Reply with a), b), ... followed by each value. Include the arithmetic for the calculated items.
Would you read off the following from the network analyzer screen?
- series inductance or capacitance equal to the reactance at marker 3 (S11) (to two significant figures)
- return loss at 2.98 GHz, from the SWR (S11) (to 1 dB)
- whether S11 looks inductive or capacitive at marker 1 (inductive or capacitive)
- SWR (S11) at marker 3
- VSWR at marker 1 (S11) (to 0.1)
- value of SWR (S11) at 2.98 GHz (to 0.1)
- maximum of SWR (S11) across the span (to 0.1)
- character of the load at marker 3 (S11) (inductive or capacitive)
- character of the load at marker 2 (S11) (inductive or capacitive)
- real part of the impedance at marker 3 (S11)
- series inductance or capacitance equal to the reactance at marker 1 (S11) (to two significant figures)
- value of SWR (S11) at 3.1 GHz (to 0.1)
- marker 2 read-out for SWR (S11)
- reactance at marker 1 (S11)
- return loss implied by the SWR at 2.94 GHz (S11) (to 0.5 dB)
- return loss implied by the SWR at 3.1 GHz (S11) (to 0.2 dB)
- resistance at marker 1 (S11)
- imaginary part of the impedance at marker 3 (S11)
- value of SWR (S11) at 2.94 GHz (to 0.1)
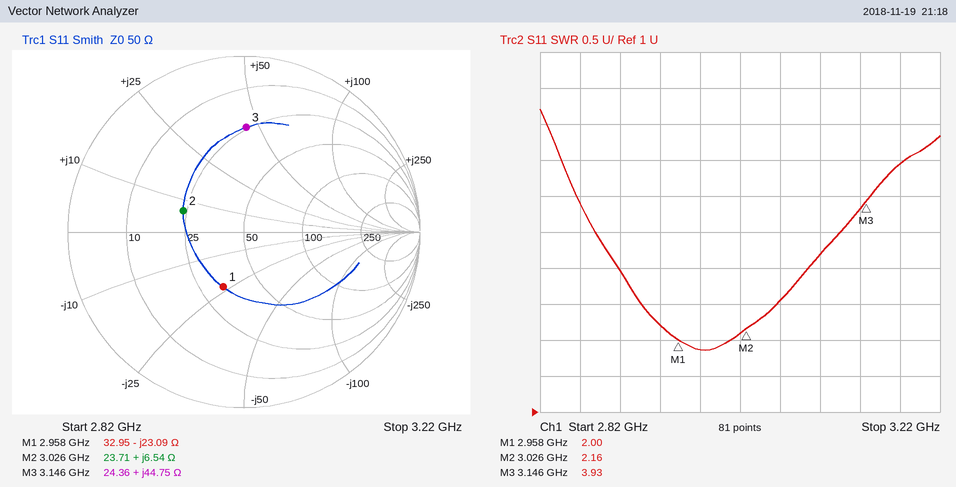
a) L = 44.75 Ω/(2π × 3.146 GHz) ≈ 2.3 nH
b) −20 log10((1.9 − 1)/(1.9 + 1)) ≈ 10 dB
c) capacitive
d) 3.93
e) 2.0
f) 1.9
g) 5.2
h) inductive
i) inductive
j) 24.36 Ω
k) C = 1/(2π × 2.958 GHz × 23.09 Ω) ≈ 2.3 pF
l) 3.2
m) 2.16
n) -23.09 Ω
o) −20 log10((2.2 − 1)/(2.2 + 1)) ≈ 8.5 dB
p) −20 log10((3.2 − 1)/(3.2 + 1)) ≈ 5.6 dB
q) 32.95 Ω
r) +44.75 Ω
s) 2.2
